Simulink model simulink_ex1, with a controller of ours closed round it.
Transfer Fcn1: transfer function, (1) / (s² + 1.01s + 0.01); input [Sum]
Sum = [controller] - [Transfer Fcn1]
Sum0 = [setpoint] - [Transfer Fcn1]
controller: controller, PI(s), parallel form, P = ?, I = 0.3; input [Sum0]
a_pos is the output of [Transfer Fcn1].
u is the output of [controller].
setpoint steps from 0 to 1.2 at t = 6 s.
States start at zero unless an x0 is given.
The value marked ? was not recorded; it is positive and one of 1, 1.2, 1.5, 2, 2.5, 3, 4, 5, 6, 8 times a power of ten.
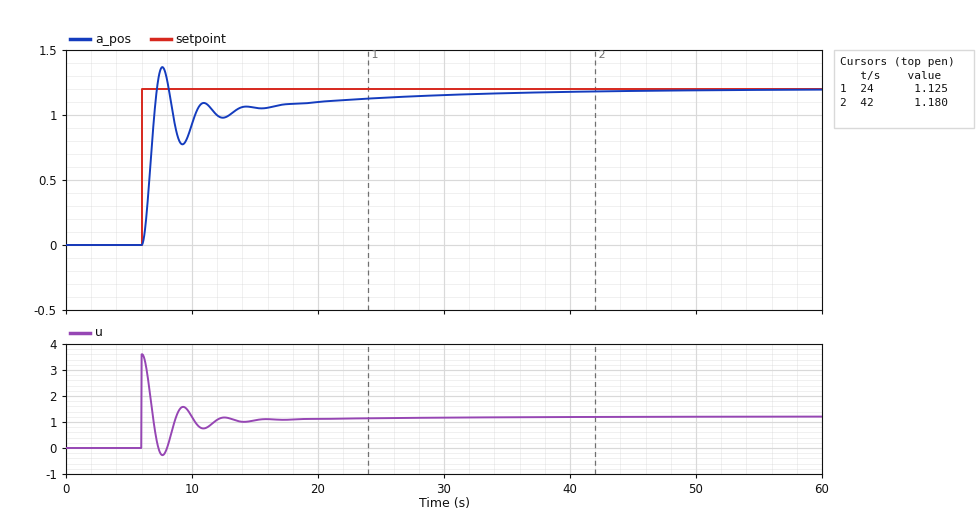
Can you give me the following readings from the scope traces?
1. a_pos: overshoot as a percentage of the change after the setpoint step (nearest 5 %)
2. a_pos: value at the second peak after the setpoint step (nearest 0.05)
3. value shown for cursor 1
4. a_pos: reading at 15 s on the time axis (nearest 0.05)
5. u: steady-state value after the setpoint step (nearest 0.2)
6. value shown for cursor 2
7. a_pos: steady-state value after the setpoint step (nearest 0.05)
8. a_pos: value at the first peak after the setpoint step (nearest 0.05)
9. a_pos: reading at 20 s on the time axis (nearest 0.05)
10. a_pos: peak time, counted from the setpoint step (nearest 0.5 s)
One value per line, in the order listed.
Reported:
15 %
1.10
1.125
1.05
1.2
1.180
1.20
1.35
1.10
1.5 s
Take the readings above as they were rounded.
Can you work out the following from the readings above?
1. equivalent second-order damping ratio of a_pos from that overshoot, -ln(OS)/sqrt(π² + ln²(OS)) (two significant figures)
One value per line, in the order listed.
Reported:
0.52
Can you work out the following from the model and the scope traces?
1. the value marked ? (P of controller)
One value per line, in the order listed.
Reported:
3
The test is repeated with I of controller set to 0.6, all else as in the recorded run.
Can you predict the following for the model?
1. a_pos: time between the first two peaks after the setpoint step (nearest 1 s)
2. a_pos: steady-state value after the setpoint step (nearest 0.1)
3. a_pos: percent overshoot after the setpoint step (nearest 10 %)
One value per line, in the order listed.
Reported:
3 s
1.2
20 %
